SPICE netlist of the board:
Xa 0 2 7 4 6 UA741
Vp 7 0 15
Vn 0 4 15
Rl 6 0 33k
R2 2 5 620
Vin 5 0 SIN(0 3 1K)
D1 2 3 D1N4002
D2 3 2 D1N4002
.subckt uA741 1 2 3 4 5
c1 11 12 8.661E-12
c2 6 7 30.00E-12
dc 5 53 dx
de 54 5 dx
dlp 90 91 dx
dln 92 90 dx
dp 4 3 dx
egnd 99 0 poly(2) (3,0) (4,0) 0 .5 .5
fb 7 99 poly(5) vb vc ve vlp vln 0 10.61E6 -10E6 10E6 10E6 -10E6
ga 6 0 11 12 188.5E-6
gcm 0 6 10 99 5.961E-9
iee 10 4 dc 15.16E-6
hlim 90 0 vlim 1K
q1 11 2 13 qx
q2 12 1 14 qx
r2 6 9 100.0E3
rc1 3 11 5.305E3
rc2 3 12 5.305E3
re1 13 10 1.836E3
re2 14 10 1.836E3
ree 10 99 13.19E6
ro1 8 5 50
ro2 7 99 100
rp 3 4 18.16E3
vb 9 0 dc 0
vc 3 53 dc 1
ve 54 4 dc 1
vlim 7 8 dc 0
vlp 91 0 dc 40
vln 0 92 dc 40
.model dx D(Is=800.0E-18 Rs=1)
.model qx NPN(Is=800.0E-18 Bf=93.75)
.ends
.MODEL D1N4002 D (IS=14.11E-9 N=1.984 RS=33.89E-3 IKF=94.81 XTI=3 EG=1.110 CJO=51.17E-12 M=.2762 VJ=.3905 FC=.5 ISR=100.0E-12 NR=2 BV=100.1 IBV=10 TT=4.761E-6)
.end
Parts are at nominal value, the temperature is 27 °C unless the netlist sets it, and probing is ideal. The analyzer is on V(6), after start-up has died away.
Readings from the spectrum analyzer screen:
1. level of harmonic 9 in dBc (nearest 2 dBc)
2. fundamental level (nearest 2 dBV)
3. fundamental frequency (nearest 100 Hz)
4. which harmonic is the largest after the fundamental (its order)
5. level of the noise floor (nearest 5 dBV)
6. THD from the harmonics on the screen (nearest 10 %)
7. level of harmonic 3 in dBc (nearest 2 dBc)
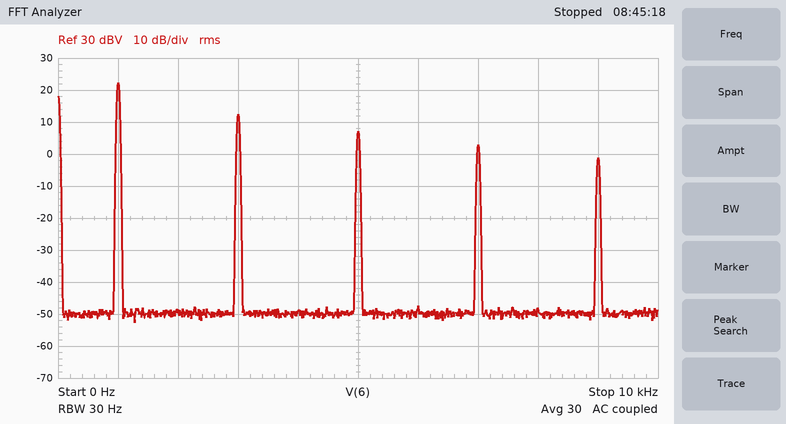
-24 dBc
22 dBV
1.0 kHz
3
-50 dBV
40 %
-10 dBc
